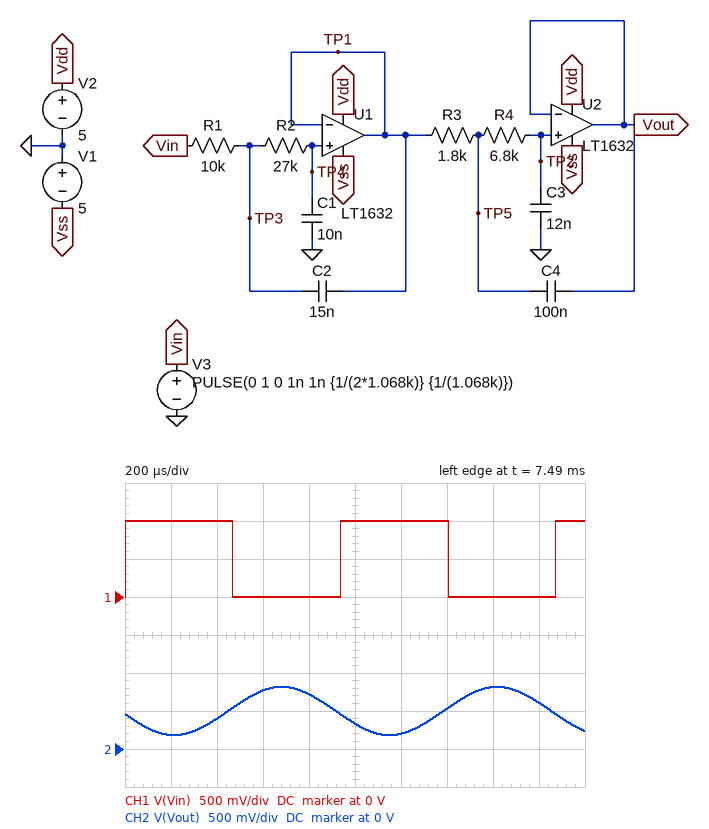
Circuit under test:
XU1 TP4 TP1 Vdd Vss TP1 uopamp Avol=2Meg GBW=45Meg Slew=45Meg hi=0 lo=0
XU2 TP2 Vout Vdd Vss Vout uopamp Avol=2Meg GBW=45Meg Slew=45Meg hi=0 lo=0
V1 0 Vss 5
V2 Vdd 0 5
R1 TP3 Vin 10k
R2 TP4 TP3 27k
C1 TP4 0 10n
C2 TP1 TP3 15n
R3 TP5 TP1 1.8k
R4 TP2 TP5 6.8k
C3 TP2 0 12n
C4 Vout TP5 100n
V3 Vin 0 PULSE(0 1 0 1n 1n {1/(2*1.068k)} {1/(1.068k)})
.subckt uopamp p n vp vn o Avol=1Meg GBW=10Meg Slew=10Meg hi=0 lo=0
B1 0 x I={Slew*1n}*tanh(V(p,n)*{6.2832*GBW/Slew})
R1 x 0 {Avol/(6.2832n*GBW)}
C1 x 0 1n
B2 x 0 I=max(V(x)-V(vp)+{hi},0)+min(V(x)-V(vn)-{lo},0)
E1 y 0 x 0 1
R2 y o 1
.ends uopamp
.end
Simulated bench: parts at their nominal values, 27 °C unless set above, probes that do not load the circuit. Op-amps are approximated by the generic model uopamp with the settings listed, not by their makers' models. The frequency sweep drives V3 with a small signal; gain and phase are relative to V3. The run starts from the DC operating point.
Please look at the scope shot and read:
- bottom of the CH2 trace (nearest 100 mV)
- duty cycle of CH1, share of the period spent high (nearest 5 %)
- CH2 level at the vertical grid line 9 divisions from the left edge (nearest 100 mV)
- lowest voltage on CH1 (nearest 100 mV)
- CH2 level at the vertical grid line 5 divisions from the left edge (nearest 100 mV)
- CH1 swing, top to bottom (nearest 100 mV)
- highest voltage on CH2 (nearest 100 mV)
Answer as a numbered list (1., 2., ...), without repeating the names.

1. 200 mV
2. 50 %
3. 600 mV
4. 0 V
5. 300 mV
6. 1.0 V
7. 800 mV
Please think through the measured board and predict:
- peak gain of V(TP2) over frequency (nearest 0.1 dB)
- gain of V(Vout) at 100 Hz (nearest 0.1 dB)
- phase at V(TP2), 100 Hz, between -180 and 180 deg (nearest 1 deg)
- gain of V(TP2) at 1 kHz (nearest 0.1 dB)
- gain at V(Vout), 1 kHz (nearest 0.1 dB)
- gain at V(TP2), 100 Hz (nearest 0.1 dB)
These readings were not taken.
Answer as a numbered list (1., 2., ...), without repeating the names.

1. 0 dB
2. -0.1 dB
3. -17 deg
4. -5.4 dB
5. -5.4 dB
6. -0.1 dB
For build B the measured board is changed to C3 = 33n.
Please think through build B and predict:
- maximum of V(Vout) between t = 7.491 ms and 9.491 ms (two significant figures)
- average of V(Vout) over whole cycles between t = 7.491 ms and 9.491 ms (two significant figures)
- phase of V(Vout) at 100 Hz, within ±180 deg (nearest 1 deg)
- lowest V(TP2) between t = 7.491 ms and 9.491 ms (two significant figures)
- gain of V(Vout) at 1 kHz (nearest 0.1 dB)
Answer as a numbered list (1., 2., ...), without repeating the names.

1. 620 mV
2. 500 mV
3. -24 deg
4. 380 mV
5. -13.1 dB
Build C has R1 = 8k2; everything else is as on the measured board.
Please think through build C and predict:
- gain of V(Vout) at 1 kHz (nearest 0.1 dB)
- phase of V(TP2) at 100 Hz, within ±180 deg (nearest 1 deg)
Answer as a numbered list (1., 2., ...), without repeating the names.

1. -4.7 dB
2. -16 deg
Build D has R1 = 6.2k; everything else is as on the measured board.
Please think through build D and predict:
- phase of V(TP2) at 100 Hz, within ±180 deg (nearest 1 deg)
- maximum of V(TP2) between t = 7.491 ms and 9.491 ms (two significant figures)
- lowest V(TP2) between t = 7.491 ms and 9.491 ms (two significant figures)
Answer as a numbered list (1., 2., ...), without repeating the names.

1. -16 deg
2. 870 mV
3. 130 mV
